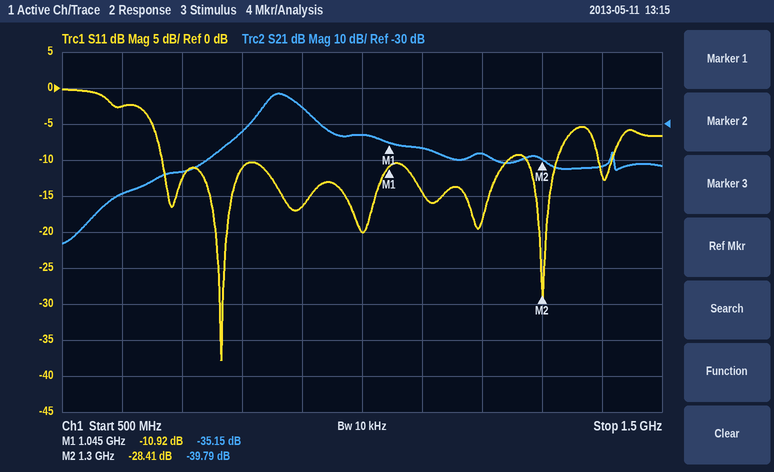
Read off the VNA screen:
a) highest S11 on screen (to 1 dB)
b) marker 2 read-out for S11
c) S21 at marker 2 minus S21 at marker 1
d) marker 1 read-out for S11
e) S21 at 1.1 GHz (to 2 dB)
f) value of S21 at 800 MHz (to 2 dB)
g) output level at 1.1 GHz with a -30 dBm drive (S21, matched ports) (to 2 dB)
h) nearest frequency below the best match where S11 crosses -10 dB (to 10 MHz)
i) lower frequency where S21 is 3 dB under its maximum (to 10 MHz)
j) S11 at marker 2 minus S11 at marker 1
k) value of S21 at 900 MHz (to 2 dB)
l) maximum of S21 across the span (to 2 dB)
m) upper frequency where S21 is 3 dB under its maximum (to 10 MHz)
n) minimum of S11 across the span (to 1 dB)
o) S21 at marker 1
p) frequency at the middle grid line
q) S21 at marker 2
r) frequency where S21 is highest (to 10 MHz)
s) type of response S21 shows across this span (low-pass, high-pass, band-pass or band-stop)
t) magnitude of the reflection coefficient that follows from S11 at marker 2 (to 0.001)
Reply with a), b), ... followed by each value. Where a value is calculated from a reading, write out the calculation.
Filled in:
a) 0 dB
b) -28.41 dB
c) -39.79 − (-35.15) = -4.64 dB
d) -10.92 dB
e) -36 dB
f) -32 dB
g) -30 dBm + (-36 dB) = -66 dBm
h) 670 MHz
i) 840 MHz
j) -28.41 − (-10.92) = -17.49 dB
k) -26 dB
l) -22 dB
m) 890 MHz
n) -38 dB
o) -35.15 dB
p) 1 GHz
q) -39.79 dB
r) 860 MHz
s) band-pass
t) 10^(-28.41/20) ≈ 0.038
